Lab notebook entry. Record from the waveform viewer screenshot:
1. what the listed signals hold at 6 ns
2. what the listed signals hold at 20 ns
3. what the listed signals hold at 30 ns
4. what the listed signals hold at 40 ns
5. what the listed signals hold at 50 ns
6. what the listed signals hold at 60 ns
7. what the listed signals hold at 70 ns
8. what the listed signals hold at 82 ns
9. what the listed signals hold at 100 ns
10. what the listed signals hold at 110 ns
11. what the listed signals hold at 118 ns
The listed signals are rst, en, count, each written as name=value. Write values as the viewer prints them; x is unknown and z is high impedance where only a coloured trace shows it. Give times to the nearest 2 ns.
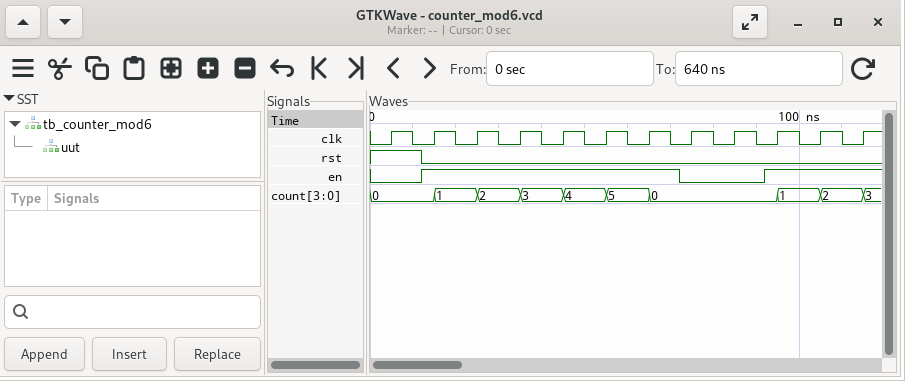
rst=1, en=0, count=0
rst=0, en=1, count=1
rst=0, en=1, count=2
rst=0, en=1, count=3
rst=0, en=1, count=4
rst=0, en=1, count=5
rst=0, en=1, count=0
rst=0, en=0, count=0
rst=0, en=1, count=1
rst=0, en=1, count=2
rst=0, en=1, count=3
